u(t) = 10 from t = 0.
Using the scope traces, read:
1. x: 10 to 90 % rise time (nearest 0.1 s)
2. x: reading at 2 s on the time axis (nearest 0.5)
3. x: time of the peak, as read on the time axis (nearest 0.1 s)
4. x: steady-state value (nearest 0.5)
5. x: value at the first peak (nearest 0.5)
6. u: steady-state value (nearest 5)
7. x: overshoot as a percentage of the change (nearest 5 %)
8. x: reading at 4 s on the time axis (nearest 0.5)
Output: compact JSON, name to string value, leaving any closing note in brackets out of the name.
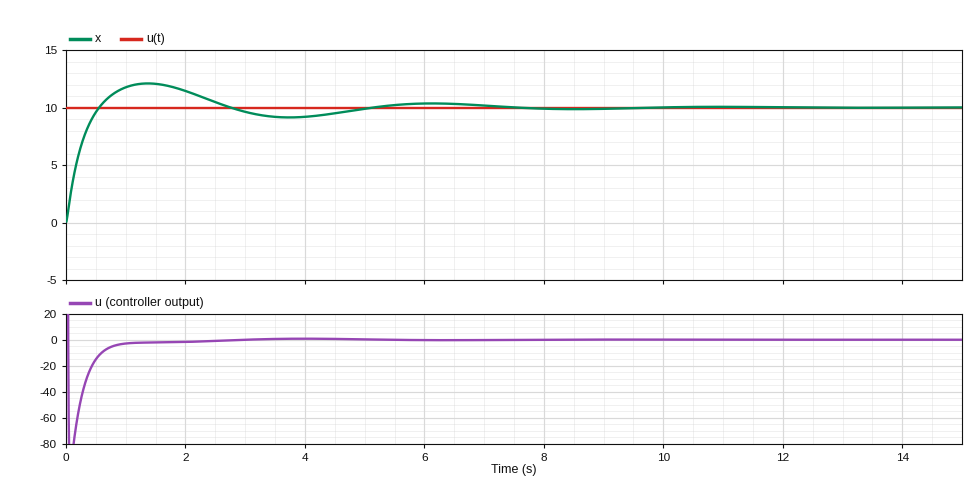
{"x: 10 to 90 % rise time": "0.4 s", "x: reading at 2 s on the time axis": "11.5", "x: time of the peak, as read on the time axis": "1.4 s", "x: steady-state value": "10.0", "x: value at the first peak": "12.0", "u: steady-state value": "0", "x: overshoot as a percentage of the change": "20 %", "x: reading at 4 s on the time axis": "9.0"}
